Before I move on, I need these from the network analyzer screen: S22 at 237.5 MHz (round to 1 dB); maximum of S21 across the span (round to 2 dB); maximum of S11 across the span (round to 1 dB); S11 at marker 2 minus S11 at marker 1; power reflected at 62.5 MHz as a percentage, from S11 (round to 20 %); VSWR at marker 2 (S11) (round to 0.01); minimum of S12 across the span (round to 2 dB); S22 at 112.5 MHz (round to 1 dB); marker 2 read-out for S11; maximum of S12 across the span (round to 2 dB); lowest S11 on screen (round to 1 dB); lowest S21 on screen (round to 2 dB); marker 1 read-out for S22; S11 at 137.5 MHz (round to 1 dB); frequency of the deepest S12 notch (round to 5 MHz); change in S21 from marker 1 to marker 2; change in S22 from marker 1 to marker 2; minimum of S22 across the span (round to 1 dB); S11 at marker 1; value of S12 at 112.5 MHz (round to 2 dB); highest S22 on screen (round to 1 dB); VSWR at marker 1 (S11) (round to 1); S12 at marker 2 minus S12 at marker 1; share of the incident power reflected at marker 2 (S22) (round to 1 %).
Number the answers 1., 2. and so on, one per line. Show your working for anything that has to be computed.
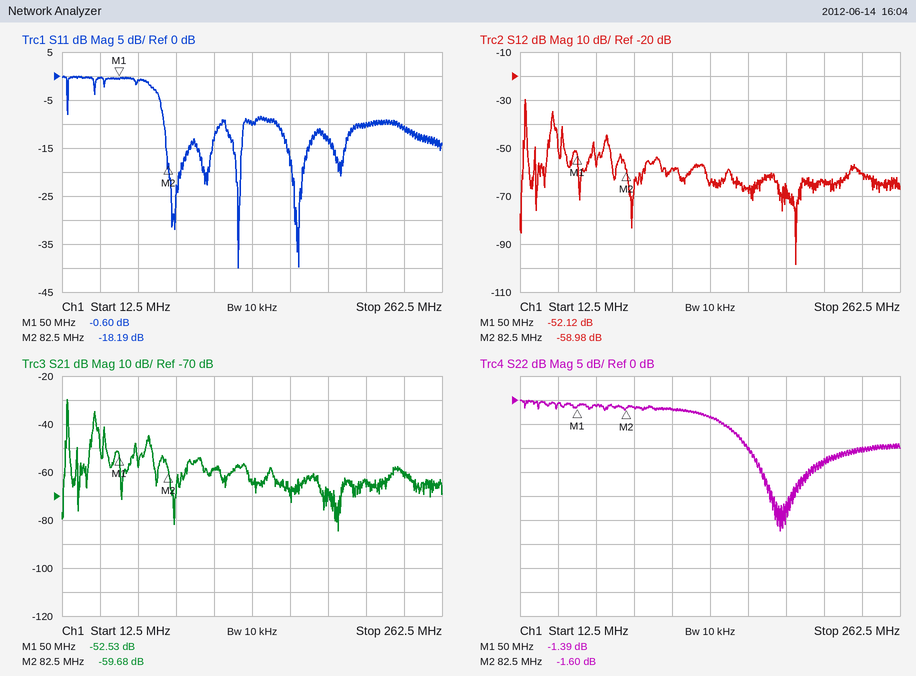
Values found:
1. -10 dB
2. -30 dB
3. 0 dB
4. -18.19 − (-0.6) = -17.59 dB
5. 10^(-1/10) ≈ 79.4 %, so 80 % to the nearest 20 %
6. (1 + 0.1232)/(1 − 0.1232) ≈ 1.28
7. -98 dB
8. -2 dB
9. -18.19 dB
10. -30 dB
11. -40 dB
12. -84 dB
13. -1.39 dB
14. -10 dB
15. 195 MHz
16. -59.68 − (-52.53) = -7.15 dB
17. -1.6 − (-1.39) = -0.21 dB
18. -27 dB
19. -0.60 dB
20. -58 dB
21. 0 dB
22. (1 + 0.9333)/(1 − 0.9333) ≈ 29
23. -58.98 − (-52.12) = -6.86 dB
24. 10^(-1.6/10) ≈ 69 %
